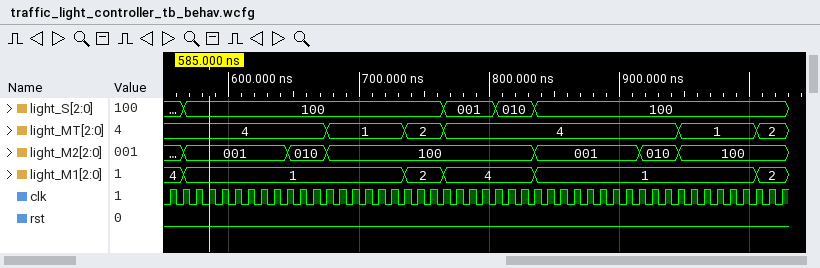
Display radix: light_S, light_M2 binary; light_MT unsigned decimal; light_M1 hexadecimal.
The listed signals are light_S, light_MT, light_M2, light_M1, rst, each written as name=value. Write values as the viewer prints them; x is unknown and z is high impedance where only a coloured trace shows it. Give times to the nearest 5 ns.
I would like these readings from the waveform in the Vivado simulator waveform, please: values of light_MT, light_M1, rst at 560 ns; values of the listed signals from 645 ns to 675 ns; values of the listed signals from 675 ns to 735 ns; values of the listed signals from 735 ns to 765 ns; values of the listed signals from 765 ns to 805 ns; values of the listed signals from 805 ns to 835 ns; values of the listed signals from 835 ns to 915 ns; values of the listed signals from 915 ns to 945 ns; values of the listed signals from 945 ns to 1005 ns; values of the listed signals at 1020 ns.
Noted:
light_MT=4, light_M1=4, rst=0
light_S=100, light_MT=4, light_M2=010, light_M1=1, rst=0
light_S=100, light_MT=1, light_M2=100, light_M1=1, rst=0
light_S=100, light_MT=2, light_M2=100, light_M1=2, rst=0
light_S=001, light_MT=4, light_M2=100, light_M1=4, rst=0
light_S=010, light_MT=4, light_M2=100, light_M1=4, rst=0
light_S=100, light_MT=4, light_M2=001, light_M1=1, rst=0
light_S=100, light_MT=4, light_M2=010, light_M1=1, rst=0
light_S=100, light_MT=1, light_M2=100, light_M1=1, rst=0
light_S=100, light_MT=2, light_M2=100, light_M1=2, rst=0
